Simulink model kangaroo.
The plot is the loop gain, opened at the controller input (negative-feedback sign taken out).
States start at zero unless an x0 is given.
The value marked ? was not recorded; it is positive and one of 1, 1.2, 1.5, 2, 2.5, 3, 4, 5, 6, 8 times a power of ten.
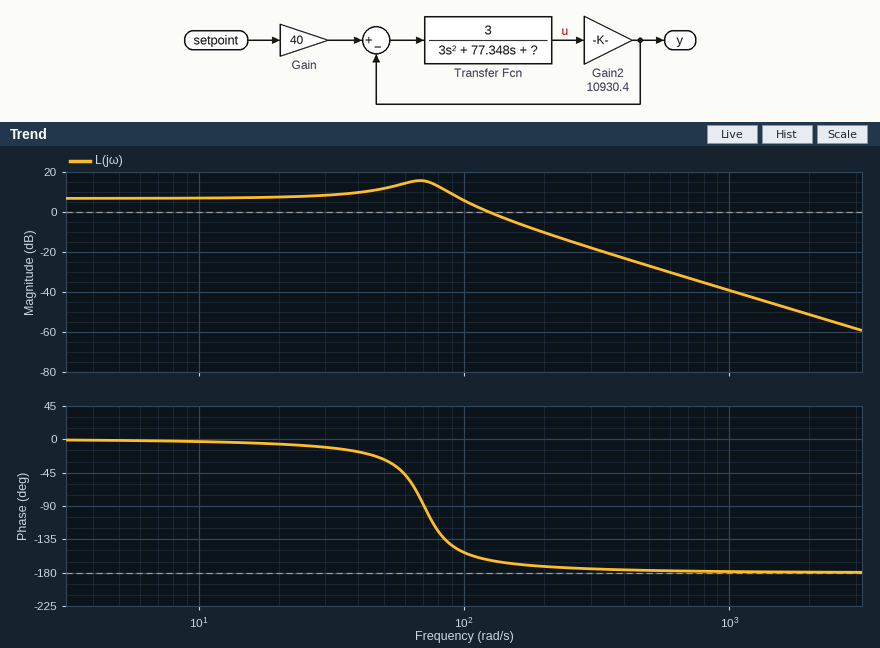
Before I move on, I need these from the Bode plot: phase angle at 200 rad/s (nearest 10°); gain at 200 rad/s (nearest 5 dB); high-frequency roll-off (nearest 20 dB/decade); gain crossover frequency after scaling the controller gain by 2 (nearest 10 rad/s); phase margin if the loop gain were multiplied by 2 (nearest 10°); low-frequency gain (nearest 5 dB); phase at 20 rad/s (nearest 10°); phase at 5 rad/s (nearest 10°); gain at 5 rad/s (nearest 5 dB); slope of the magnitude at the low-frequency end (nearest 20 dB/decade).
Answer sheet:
-170°
-10 dB
-40 dB/decade
160 rad/s
10°
5 dB
-10°
0°
5 dB
0 dB/decade
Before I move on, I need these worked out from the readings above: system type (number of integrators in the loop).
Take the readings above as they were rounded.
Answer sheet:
0
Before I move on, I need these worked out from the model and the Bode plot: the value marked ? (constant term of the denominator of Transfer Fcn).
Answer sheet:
15000
